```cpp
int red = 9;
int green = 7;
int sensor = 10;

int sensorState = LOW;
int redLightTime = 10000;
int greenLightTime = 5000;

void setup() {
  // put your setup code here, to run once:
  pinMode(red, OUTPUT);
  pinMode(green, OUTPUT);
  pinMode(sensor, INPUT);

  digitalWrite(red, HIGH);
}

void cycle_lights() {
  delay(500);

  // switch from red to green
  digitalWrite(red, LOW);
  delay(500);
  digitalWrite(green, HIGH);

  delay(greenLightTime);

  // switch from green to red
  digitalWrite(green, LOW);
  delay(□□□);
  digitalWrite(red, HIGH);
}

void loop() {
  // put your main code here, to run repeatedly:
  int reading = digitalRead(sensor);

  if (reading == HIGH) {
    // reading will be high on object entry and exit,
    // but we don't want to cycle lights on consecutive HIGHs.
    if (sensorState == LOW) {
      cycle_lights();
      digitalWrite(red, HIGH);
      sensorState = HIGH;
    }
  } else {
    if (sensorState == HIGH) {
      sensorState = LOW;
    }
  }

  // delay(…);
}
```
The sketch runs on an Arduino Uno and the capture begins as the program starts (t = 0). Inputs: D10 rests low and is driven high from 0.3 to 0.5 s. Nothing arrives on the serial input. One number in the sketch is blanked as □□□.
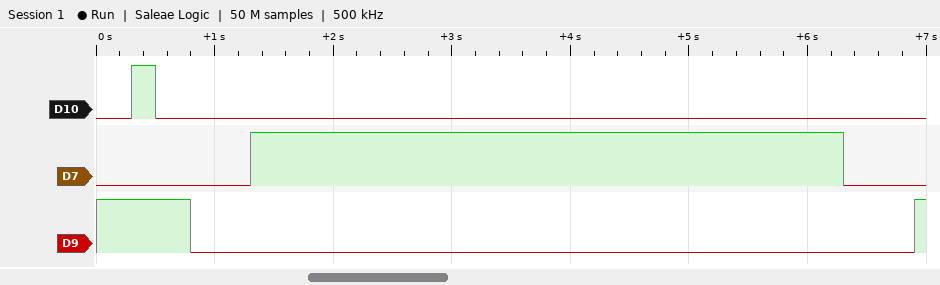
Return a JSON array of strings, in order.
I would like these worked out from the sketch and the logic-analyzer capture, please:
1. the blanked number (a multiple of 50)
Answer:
["600"]
